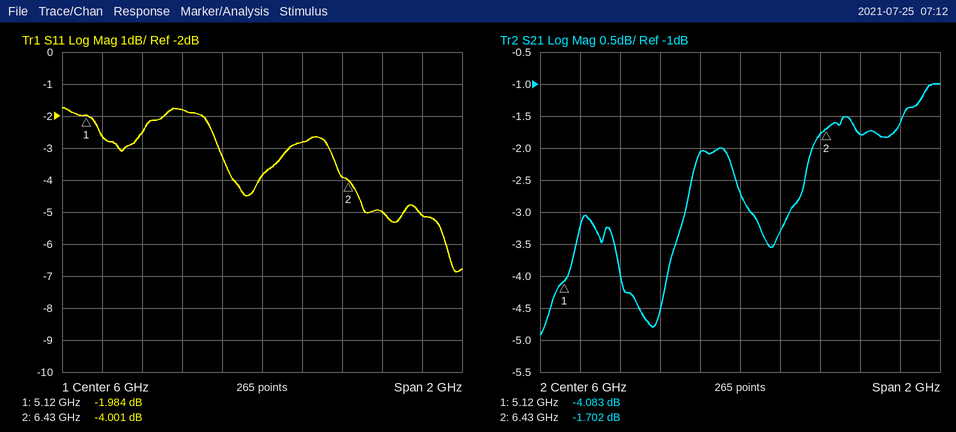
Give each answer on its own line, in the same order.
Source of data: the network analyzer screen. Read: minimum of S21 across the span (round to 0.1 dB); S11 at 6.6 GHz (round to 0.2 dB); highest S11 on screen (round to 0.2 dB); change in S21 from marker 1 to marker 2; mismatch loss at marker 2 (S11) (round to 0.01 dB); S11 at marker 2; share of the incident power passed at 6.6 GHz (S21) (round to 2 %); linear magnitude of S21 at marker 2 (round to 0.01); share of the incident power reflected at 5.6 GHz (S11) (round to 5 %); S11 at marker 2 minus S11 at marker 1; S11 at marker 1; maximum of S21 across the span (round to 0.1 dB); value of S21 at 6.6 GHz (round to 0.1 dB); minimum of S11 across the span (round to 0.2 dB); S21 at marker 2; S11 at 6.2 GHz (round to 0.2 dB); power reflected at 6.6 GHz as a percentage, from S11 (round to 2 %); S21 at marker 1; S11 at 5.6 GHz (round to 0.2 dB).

-4.9 dB
-5.0 dB
-1.8 dB
2.381 dB
2.20 dB
-4.001 dB
66 %
0.82
65 %
-2.017 dB
-1.984 dB
-1.0 dB
-1.8 dB
-6.8 dB
-1.702 dB
-2.8 dB
32 %
-4.083 dB
-1.8 dB
